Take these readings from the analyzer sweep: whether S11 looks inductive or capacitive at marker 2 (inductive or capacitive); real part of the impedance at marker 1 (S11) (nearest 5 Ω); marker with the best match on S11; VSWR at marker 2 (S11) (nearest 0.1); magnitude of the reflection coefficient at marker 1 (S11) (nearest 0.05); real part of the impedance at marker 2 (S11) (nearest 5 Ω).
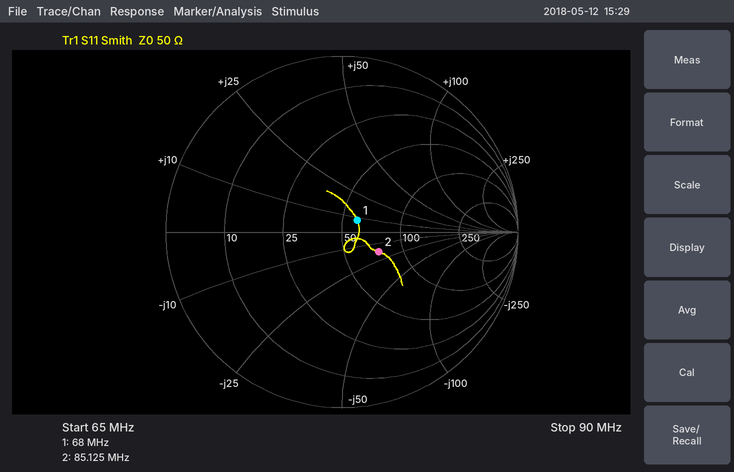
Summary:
capacitive
60 Ω
marker 1
1.6
0.10
75 Ω
